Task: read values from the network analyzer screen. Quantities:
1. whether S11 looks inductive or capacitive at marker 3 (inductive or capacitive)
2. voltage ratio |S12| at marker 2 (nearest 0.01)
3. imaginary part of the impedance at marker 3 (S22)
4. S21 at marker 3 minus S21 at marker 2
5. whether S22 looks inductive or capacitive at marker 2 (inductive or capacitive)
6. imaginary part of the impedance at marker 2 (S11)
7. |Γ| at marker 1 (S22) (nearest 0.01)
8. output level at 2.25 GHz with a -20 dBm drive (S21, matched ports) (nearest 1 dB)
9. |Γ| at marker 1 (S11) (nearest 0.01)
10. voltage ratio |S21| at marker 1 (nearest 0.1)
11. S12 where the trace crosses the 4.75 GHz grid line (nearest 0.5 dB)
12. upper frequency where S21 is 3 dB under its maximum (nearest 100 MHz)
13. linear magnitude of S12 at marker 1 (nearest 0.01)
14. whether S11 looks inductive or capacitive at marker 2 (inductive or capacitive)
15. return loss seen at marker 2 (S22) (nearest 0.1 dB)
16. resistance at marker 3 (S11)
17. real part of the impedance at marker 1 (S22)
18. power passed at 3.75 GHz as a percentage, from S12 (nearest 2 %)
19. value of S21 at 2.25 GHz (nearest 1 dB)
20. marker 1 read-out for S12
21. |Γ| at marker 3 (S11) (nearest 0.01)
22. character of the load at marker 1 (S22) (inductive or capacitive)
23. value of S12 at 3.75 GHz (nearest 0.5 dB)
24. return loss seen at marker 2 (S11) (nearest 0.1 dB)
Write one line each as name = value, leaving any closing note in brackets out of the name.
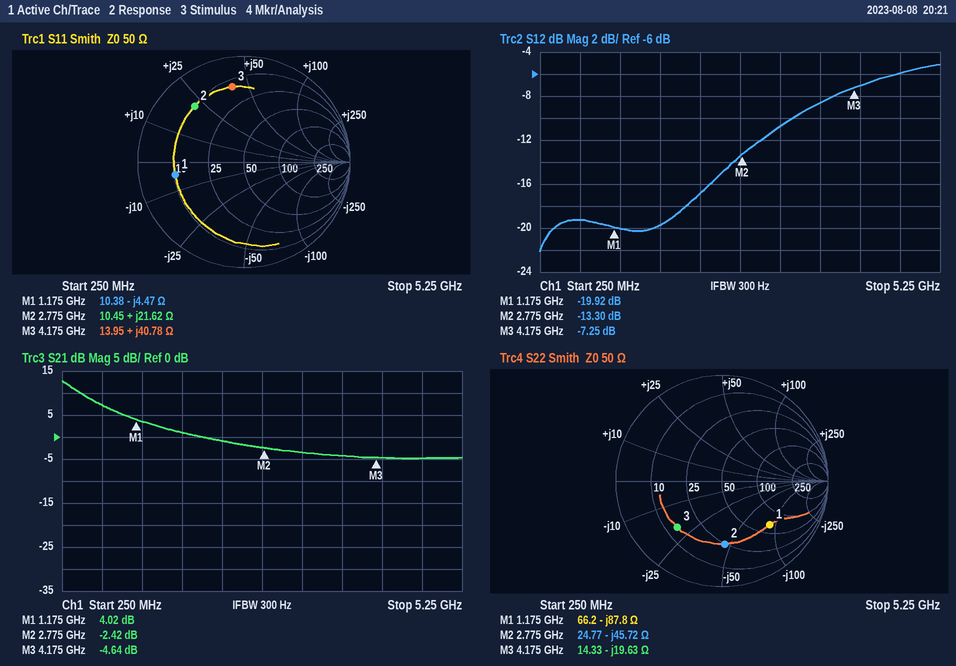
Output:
whether S11 looks inductive or capacitive at marker 3 = inductive
voltage ratio |S12| at marker 2 = 0.22
imaginary part of the impedance at marker 3 = -19.63 Ω
S21 at marker 3 minus S21 at marker 2 = -2.22 dB
whether S22 looks inductive or capacitive at marker 2 = capacitive
imaginary part of the impedance at marker 2 = +21.62 Ω
|Γ| at marker 1 (S22) = 0.61
output level at 2.25 GHz with a -20 dBm drive (S21, matched ports) = -21 dBm
|Γ| at marker 1 (S11) = 0.66
voltage ratio |S21| at marker 1 = 1.6
S12 where the trace crosses the 4.75 GHz grid line = -6.0 dB
upper frequency where S21 is 3 dB under its maximum = 500 MHz
linear magnitude of S12 at marker 1 = 0.10
whether S11 looks inductive or capacitive at marker 2 = inductive
return loss seen at marker 2 (S22) = 4.5 dB
resistance at marker 3 = 13.95 Ω
real part of the impedance at marker 1 = 66.2 Ω
power passed at 3.75 GHz as a percentage, from S12 = 14 %
value of S21 at 2.25 GHz = -1 dB
marker 1 read-out for S12 = -19.92 dB
|Γ| at marker 3 (S11) = 0.72
character of the load at marker 1 (S22) = capacitive
value of S12 at 3.75 GHz = -8.5 dB
return loss seen at marker 2 (S11) = 3.1 dB
